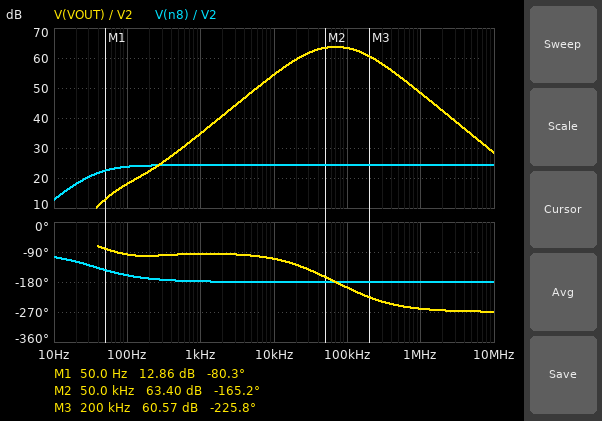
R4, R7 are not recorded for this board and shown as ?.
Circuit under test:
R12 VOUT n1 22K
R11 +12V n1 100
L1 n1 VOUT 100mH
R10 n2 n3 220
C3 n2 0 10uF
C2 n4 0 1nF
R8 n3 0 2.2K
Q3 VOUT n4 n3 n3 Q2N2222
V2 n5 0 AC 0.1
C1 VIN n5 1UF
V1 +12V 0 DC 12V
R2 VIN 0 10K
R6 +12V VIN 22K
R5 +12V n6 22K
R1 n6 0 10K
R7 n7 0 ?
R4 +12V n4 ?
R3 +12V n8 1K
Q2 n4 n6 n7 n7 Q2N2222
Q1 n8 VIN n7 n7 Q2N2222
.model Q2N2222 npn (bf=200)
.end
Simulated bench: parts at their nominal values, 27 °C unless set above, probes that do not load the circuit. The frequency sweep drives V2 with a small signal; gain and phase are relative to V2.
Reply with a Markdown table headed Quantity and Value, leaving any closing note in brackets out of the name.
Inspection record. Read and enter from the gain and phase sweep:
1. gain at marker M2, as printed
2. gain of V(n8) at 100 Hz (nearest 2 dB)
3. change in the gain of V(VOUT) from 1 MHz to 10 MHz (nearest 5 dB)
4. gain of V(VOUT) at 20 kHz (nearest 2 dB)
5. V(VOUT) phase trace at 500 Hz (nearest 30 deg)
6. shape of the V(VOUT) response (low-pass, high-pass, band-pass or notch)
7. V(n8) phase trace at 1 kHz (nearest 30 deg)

| Quantity | Value |
|---|---|
| gain at marker M2, as printed | 63.40 dB |
| gain of V(n8) at 100 Hz | 24 dB |
| change in the gain of V(VOUT) from 1 MHz to 10 MHz | -20 dB |
| gain of V(VOUT) at 20 kHz | 60 dB |
| V(VOUT) phase trace at 500 Hz | -90 deg |
| shape of the V(VOUT) response | band-pass |
| V(n8) phase trace at 1 kHz | -180 deg |
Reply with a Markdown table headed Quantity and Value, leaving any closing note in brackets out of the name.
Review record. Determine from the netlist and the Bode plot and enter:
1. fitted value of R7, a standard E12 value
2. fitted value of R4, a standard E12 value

| Quantity | Value |
|---|---|
| fitted value of R7, a standard E12 value | 820 Ω |
| fitted value of R4, a standard E12 value | 1.2 kΩ |
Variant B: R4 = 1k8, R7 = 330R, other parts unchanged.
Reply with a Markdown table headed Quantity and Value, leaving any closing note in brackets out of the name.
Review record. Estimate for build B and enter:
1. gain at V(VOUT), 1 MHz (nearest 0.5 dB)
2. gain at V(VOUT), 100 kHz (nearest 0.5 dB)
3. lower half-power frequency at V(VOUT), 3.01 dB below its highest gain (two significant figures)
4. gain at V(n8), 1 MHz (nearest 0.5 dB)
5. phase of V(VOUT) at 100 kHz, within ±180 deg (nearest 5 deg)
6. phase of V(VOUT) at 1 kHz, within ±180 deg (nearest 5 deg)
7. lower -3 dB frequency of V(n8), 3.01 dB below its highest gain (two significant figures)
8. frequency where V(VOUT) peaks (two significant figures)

| Quantity | Value |
|---|---|
| gain at V(VOUT), 1 MHz | 50.5 dB |
| gain at V(VOUT), 100 kHz | 67.5 dB |
| lower half-power frequency at V(VOUT), 3.01 dB below its highest gain | 22 kHz |
| gain at V(n8), 1 MHz | 27.5 dB |
| phase of V(VOUT) at 100 kHz, within ±180 deg | 150 deg |
| phase of V(VOUT) at 1 kHz, within ±180 deg | -95 deg |
| lower -3 dB frequency of V(n8), 3.01 dB below its highest gain | 42 Hz |
| frequency where V(VOUT) peaks | 57 kHz |
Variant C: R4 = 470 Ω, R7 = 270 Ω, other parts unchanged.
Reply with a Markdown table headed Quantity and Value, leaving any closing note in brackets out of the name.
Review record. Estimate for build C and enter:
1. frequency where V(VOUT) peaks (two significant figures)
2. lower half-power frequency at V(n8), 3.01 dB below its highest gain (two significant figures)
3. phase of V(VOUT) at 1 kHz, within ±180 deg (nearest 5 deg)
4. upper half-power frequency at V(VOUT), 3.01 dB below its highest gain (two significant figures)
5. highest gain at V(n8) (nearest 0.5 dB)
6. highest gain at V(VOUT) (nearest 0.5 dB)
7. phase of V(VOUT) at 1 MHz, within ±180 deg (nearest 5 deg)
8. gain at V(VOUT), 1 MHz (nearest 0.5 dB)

| Quantity | Value |
|---|---|
| frequency where V(VOUT) peaks | 110 kHz |
| lower half-power frequency at V(n8), 3.01 dB below its highest gain | 43 Hz |
| phase of V(VOUT) at 1 kHz, within ±180 deg | -95 deg |
| upper half-power frequency at V(VOUT), 3.01 dB below its highest gain | 410 kHz |
| highest gain at V(n8) | 28.0 dB |
| highest gain at V(VOUT) | 60.0 dB |
| phase of V(VOUT) at 1 MHz, within ±180 deg | 110 deg |
| gain at V(VOUT), 1 MHz | 51.0 dB |
